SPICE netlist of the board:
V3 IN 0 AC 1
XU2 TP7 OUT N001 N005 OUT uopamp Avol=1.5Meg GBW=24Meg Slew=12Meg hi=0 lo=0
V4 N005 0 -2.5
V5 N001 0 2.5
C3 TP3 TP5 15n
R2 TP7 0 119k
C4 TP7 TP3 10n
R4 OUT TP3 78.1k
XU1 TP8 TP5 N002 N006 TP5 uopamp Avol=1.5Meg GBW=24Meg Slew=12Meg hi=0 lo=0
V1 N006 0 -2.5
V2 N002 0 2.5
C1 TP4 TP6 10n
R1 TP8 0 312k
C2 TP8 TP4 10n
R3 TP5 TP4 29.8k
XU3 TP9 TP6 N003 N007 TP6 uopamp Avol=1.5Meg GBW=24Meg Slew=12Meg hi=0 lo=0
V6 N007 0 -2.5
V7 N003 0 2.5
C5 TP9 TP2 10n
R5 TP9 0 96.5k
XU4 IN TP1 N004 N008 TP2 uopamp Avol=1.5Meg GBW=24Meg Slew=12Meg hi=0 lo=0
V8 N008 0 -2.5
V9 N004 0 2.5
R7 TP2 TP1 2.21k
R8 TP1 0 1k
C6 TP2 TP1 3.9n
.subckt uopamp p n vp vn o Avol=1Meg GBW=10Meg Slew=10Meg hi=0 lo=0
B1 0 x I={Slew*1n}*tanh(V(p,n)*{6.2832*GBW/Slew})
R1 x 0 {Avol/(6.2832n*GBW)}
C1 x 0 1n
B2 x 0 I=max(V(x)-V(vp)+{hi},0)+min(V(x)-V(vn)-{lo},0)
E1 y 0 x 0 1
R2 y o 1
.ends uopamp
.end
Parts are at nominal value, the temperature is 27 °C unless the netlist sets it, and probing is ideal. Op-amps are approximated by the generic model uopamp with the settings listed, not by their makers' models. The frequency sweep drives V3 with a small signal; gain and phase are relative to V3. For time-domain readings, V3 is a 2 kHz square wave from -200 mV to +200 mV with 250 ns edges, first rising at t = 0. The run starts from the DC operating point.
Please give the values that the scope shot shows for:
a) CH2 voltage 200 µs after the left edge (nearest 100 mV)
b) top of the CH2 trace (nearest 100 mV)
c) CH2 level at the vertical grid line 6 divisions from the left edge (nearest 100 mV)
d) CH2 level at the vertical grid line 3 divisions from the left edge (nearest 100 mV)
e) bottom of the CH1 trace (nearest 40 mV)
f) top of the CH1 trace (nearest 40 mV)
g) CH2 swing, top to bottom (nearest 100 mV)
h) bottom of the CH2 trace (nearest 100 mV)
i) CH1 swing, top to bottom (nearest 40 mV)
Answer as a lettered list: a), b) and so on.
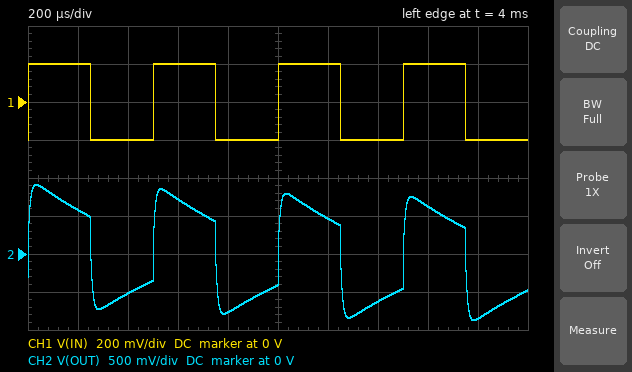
a) 600 mV
b) 900 mV
c) 500 mV
d) 700 mV
e) -200 mV
f) 200 mV
g) 1.8 V
h) -900 mV
i) 400 mV
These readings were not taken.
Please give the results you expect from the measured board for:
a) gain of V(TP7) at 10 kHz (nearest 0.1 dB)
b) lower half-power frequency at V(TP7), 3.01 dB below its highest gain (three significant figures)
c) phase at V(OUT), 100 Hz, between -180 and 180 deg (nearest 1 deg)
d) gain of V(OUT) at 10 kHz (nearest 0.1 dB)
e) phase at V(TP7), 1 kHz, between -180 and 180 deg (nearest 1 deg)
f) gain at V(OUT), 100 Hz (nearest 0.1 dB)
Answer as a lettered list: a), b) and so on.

a) 9.1 dB
b) 159 Hz
c) -42 deg
d) 9.1 dB
e) 26 deg
f) -9.1 dB
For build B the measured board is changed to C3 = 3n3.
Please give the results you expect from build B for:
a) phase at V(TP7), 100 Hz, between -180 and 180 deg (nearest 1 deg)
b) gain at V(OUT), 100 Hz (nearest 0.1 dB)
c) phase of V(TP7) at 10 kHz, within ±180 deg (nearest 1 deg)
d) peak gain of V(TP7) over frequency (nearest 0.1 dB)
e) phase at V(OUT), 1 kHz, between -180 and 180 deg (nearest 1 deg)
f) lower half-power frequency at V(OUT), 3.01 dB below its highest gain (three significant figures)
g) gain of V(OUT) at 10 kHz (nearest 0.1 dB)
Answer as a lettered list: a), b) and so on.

a) -9 deg
b) -20.7 dB
c) -14 deg
d) 10.0 dB
e) 44 deg
f) 353 Hz
g) 9.1 dB
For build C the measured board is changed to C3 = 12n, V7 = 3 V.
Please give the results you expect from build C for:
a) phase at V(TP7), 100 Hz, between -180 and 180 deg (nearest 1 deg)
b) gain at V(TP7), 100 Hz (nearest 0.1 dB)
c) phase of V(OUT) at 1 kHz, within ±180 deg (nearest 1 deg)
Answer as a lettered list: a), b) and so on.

a) -35 deg
b) -10.4 dB
c) 27 deg
